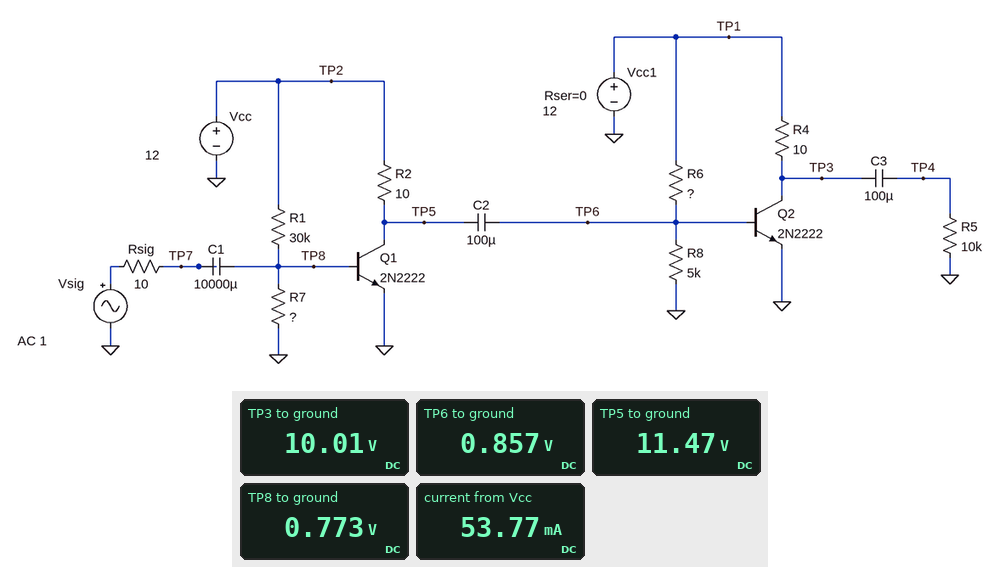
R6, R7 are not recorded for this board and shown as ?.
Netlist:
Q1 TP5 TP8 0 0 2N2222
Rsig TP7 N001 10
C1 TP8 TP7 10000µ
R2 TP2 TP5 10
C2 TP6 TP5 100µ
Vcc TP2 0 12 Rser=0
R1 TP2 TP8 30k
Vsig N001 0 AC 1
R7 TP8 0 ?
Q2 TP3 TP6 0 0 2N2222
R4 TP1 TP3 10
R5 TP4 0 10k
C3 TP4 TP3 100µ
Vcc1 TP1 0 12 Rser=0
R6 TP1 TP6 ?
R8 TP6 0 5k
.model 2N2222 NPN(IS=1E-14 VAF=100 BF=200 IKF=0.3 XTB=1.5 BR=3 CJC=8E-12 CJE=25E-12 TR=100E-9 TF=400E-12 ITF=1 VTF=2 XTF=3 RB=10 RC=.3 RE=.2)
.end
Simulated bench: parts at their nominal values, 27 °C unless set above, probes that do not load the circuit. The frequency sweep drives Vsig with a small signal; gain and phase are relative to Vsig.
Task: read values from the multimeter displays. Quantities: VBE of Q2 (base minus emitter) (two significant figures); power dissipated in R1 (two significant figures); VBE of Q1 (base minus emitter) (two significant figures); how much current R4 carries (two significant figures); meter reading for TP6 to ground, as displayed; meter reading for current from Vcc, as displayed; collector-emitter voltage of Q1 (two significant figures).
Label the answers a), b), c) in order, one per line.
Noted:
a) 860 mV
b) 4.2 mW
c) 770 mV
d) 200 mA
e) 0.857 V
f) 53.77 mA
g) 11 V
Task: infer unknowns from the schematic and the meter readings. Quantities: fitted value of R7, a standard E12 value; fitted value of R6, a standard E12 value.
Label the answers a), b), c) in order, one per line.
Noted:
a) 8.2 kΩ
b) 6.8 kΩ
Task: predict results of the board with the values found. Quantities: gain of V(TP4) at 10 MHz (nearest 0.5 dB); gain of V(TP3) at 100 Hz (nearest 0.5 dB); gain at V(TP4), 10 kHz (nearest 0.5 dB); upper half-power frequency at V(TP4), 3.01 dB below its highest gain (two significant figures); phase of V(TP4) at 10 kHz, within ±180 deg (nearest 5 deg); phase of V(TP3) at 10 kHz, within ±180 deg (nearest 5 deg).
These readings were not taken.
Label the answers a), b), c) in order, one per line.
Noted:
a) 41.0 dB
b) 45.5 dB
c) 45.5 dB
d) 7.8 MHz
e) 0 deg
f) 0 deg
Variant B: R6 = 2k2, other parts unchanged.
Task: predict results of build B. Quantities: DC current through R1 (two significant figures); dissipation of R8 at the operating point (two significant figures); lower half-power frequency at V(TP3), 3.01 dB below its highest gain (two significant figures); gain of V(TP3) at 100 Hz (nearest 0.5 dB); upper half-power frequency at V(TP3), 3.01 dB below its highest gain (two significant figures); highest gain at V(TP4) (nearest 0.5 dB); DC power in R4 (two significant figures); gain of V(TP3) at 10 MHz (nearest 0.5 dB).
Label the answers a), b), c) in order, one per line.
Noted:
a) 370 µA
b) 190 µW
c) 44 Hz
d) 44.0 dB
e) 7.3 MHz
f) 44.5 dB
g) 1.9 W
h) 39.5 dB
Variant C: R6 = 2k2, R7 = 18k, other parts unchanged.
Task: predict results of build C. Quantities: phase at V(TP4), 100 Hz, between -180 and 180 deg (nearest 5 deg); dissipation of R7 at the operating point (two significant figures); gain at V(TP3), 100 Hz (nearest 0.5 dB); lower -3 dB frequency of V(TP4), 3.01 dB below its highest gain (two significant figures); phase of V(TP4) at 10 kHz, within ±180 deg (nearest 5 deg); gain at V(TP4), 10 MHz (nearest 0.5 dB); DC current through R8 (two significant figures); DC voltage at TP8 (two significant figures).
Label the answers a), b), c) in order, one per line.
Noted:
a) 25 deg
b) 34 µW
c) 44.5 dB
d) 44 Hz
e) 0 deg
f) 40.0 dB
g) 190 µA
h) 780 mV
